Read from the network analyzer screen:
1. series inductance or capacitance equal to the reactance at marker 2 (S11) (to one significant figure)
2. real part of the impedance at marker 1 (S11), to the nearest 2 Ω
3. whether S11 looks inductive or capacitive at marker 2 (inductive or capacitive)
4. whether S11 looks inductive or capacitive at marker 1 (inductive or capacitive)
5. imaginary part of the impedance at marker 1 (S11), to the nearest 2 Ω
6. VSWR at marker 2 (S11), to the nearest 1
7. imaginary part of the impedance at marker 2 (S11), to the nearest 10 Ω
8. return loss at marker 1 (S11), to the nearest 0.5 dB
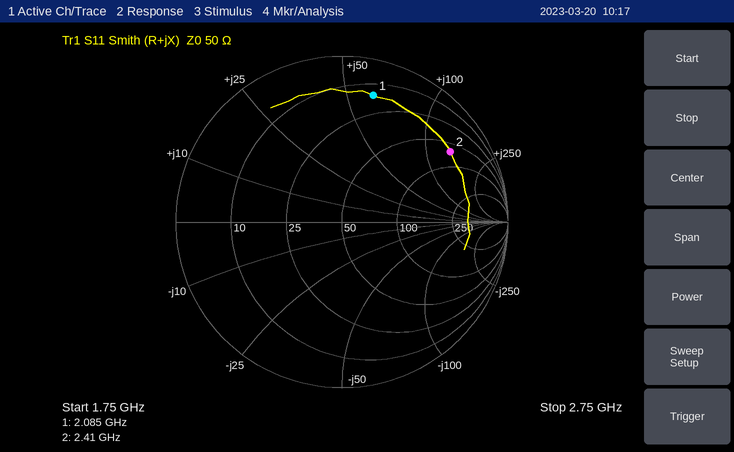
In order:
9 nH
16 Ω
inductive
inductive
+62 Ω
8
+140 Ω
2.0 dB
